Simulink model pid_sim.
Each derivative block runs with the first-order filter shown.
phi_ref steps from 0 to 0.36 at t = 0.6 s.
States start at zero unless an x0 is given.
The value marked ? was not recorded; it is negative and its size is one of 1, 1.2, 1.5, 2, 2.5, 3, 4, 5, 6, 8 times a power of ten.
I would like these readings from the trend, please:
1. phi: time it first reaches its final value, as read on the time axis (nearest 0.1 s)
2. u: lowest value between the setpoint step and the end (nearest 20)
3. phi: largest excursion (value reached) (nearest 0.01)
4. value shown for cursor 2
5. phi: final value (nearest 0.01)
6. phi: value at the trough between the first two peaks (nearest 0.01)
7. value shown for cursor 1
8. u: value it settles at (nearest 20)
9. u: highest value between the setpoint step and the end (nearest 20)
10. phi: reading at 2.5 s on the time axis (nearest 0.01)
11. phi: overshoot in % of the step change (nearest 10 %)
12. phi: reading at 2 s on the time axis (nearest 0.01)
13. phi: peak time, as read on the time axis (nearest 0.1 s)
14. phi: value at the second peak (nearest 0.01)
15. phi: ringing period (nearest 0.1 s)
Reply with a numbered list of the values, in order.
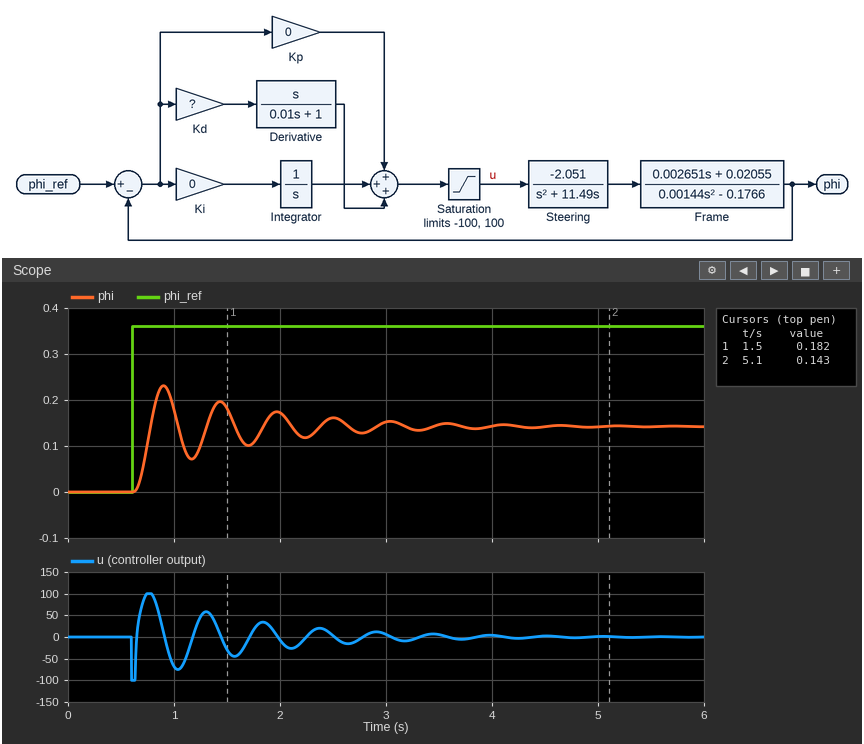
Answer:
1. 0.8 s
2. -100
3. 0.23
4. 0.143
5. 0.14
6. 0.07
7. 0.182
8. 0
9. 100
10. 0.16
11. 60 %
12. 0.17
13. 0.9 s
14. 0.20
15. 0.5 s
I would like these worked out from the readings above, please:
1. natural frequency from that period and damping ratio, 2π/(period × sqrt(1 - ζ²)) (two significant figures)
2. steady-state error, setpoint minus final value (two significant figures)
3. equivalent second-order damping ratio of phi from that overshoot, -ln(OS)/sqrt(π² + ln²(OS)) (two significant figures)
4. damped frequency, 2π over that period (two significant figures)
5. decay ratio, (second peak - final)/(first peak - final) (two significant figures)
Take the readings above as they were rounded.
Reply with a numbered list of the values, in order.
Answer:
1. 13 rad/s
2. 0.22
3. 0.16
4. 13 rad/s
5. 0.67
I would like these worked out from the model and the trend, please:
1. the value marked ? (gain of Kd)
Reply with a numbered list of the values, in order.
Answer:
1. -80
